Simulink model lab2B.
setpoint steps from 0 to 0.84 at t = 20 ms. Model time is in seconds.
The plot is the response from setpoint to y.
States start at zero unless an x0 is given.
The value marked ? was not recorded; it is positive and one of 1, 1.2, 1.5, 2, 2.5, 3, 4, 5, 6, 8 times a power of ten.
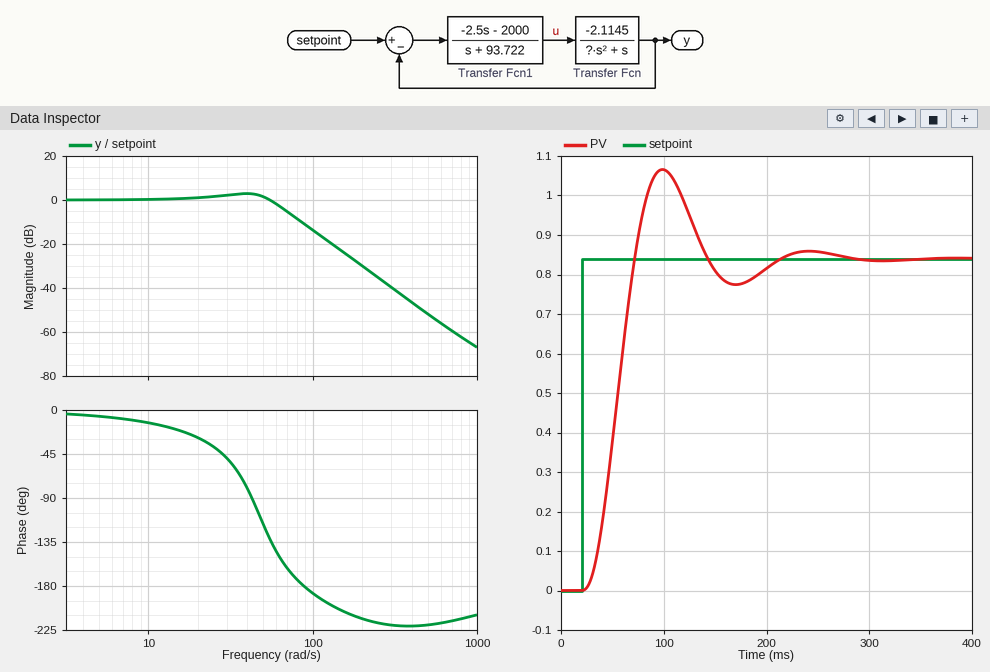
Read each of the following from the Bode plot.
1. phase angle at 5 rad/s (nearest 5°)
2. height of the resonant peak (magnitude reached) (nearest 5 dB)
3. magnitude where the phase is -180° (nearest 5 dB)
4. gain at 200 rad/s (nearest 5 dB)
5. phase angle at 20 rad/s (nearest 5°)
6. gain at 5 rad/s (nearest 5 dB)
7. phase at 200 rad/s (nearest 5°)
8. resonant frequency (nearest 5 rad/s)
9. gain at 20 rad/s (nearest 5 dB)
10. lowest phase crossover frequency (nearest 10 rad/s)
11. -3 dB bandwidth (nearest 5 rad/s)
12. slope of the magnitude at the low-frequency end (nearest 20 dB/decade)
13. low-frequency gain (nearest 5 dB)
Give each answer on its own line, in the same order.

-5°
5 dB
-10 dB
-30 dB
-30°
0 dB
-215°
40 rad/s
0 dB
90 rad/s
65 rad/s
0 dB/decade
0 dB
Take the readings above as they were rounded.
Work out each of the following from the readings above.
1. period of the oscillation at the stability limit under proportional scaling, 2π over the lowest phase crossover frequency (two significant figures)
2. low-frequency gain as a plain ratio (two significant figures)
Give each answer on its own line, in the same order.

0.070 s
1.0
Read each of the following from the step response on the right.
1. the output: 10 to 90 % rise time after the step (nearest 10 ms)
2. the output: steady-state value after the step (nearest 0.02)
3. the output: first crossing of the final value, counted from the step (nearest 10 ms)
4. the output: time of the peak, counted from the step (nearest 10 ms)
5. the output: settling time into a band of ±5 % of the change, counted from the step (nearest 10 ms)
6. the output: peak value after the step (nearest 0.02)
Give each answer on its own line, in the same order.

30 ms
0.84
50 ms
80 ms
170 ms
1.06
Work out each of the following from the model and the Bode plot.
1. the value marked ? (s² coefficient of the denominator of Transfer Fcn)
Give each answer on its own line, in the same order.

0.015
